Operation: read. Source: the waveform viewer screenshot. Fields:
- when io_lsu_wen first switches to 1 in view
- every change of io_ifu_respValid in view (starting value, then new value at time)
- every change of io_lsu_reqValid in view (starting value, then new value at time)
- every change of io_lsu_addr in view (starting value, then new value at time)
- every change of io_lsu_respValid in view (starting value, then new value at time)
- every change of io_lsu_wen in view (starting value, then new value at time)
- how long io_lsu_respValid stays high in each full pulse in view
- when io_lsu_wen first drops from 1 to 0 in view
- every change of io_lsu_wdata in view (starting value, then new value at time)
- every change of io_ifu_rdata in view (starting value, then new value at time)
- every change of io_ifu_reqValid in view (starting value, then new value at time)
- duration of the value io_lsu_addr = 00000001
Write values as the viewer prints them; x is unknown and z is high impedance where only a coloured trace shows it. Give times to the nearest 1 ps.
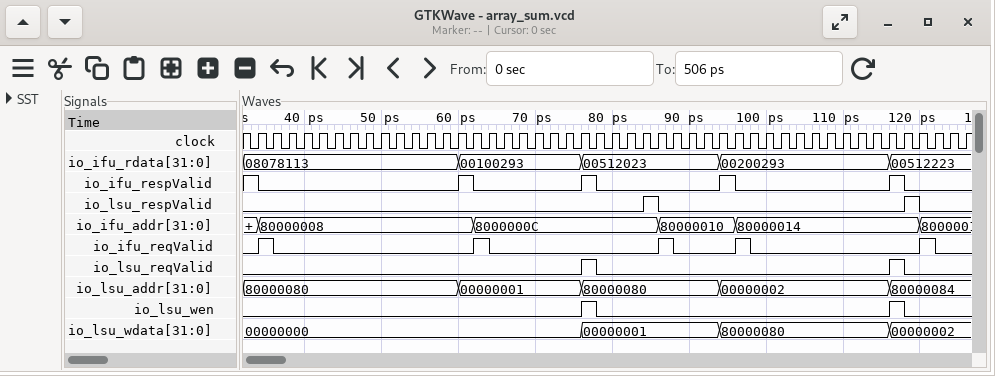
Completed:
76 ps
1, 0 at 34 ps, 1 at 60 ps, 0 at 62 ps, 1 at 76 ps, 0 at 78 ps, 1 at 94 ps, 0 at 96 ps, 1 at 116 ps, 0 at 118 ps
0, 1 at 76 ps, 0 at 78 ps, 1 at 116 ps, 0 at 118 ps
80000080, 00000001 at 60 ps, 80000080 at 76 ps, 00000002 at 94 ps, 80000084 at 116 ps
0, 1 at 84 ps, 0 at 86 ps, 1 at 118 ps, 0 at 120 ps
0, 1 at 76 ps, 0 at 78 ps, 1 at 116 ps, 0 at 118 ps
2 ps, 2 ps
78 ps
00000000, 00000001 at 76 ps, 80000080 at 94 ps, 00000002 at 116 ps
08078113, 00100293 at 60 ps, 00512023 at 76 ps, 00200293 at 94 ps, 00512223 at 116 ps
0, 1 at 34 ps, 0 at 36 ps, 1 at 62 ps, 0 at 64 ps, 1 at 86 ps, 0 at 88 ps, 1 at 96 ps, 0 at 98 ps, 1 at 120 ps, 0 at 122 ps
16 ps
